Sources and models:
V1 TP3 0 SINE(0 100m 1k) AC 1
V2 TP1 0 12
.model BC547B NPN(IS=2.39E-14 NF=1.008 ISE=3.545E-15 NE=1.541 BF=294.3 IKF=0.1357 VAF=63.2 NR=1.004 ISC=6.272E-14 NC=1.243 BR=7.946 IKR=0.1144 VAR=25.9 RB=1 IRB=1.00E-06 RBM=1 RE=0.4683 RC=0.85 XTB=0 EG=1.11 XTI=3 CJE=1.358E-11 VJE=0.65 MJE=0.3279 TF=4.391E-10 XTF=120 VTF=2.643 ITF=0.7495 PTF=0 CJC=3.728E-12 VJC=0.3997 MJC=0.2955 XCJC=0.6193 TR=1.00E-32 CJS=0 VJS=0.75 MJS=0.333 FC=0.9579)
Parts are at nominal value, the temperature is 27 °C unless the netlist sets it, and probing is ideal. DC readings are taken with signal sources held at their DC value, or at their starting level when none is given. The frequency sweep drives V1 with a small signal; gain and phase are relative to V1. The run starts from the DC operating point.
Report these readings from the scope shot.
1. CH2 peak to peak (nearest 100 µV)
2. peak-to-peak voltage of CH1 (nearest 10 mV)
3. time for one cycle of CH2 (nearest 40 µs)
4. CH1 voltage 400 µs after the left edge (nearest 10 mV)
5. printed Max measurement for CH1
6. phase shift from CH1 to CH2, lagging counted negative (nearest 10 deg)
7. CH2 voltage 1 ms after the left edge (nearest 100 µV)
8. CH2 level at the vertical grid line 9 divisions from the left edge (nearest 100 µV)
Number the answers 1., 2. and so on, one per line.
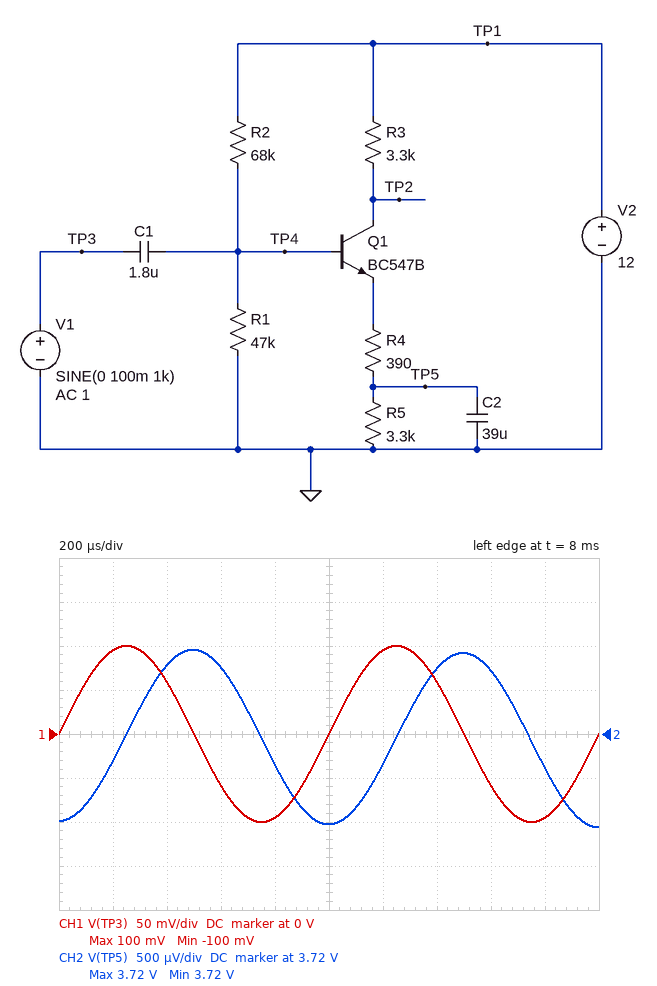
1. 2.0 mV
2. 200 mV
3. 1.00 ms
4. 60 mV
5. 100 mV
6. -90 deg
7. 3.7190 V
8. 3.7196 V
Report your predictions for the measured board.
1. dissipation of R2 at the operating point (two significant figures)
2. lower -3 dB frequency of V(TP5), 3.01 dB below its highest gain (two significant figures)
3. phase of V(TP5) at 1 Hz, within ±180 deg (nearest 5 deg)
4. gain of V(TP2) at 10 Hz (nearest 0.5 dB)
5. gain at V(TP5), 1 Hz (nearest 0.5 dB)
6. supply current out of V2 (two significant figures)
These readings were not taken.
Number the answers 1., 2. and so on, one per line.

1. 760 µW
2. 2.1 Hz
3. 65 deg
4. 14.0 dB
5. -12.0 dB
6. 1.2 mA
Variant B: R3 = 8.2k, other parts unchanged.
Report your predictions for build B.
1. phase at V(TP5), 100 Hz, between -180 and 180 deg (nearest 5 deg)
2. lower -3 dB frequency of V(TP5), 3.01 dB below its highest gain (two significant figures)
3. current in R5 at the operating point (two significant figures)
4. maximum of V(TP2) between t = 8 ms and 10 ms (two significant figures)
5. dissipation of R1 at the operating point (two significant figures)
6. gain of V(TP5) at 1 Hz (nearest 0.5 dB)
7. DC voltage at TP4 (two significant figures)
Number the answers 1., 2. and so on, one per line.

1. -30 deg
2. 1.7 Hz
3. 1.0 mA
4. 6.6 V
5. 410 µW
6. -32.5 dB
7. 4.4 V
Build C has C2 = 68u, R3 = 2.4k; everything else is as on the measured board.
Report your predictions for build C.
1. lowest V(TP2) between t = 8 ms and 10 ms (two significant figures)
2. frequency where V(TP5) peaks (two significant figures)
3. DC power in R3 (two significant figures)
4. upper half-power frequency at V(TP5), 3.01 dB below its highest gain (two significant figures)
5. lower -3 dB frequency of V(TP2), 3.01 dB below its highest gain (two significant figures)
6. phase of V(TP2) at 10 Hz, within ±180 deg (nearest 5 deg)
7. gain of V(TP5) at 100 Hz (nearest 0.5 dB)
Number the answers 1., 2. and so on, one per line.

1. 8.7 V
2. 4.6 Hz
3. 3.0 mW
4. 12 Hz
5. 8.3 Hz
6. -130 deg
7. -25.0 dB
